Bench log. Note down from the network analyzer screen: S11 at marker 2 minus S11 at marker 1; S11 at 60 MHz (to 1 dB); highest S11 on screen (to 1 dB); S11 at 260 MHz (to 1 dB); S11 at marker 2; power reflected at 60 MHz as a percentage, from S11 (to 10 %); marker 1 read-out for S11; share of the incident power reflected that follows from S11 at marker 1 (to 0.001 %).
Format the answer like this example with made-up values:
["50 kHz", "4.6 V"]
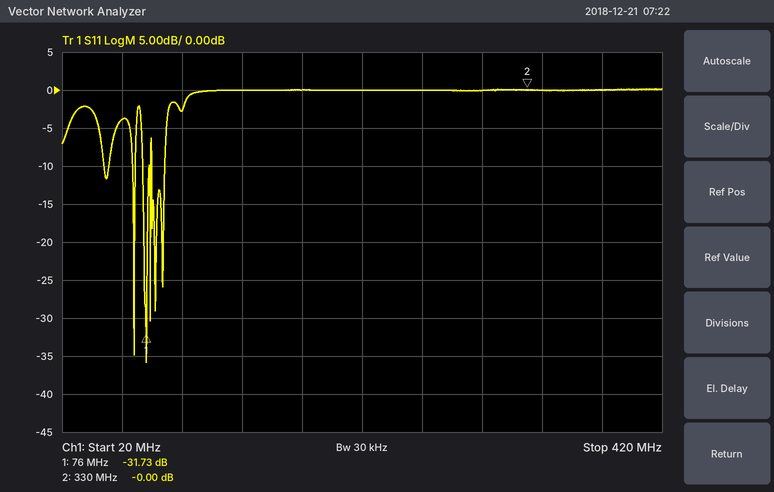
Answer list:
["31.73 dB", "-4 dB", "0 dB", "0 dB", "-0.00 dB", "40 %", "-31.73 dB", "0.067 %"]
